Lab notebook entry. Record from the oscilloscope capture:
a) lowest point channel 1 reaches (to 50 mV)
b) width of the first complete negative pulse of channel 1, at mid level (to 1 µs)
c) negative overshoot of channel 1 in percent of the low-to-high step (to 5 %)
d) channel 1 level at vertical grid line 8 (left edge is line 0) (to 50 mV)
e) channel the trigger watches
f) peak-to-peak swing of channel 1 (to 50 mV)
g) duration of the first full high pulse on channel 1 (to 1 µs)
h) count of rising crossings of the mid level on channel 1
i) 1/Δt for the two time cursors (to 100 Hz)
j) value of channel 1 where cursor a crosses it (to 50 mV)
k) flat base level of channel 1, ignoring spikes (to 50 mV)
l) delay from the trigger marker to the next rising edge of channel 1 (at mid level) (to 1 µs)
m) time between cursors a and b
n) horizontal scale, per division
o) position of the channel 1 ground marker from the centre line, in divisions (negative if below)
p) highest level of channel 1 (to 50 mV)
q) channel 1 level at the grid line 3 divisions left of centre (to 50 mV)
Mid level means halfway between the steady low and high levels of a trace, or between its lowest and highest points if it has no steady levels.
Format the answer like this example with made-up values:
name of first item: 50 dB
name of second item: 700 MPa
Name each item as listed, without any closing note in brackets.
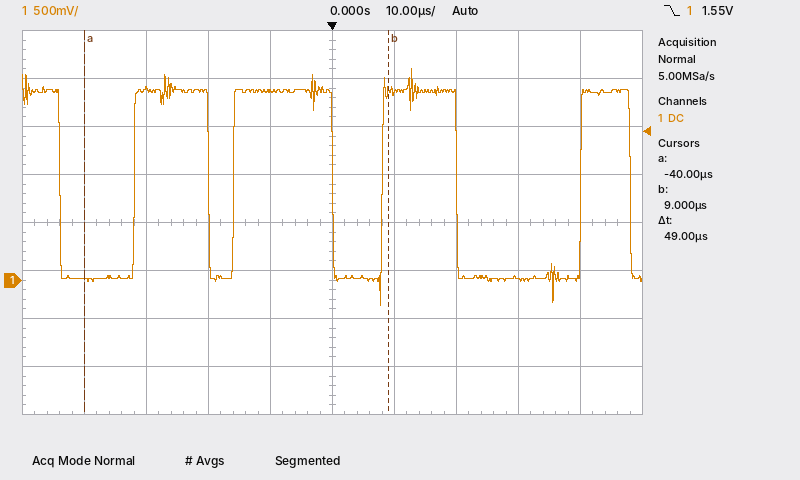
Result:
lowest point channel 1 reaches: -250 mV
width of the first complete negative pulse of channel 1, at mid level: 12 µs
negative overshoot of channel 1 in percent of the low-to-high step: 15 %
channel 1 level at vertical grid line 8 (left edge is line 0): 0 mV
channel the trigger watches: channel 1
peak-to-peak swing of channel 1: 2.45 V
duration of the first full high pulse on channel 1: 12 µs
count of rising crossings of the mid level on channel 1: 4
1/Δt for the two time cursors: 20.4 kHz
value of channel 1 where cursor a crosses it: 0 mV
flat base level of channel 1, ignoring spikes: 0 mV
delay from the trigger marker to the next rising edge of channel 1 (at mid level): 8 µs
time between cursors a and b: 49 µs
horizontal scale, per division: 10 µs
position of the channel 1 ground marker from the centre line, in divisions: -1.2 div
highest level of channel 1: 2.20 V
channel 1 level at the grid line 3 divisions left of centre: 2.00 V
